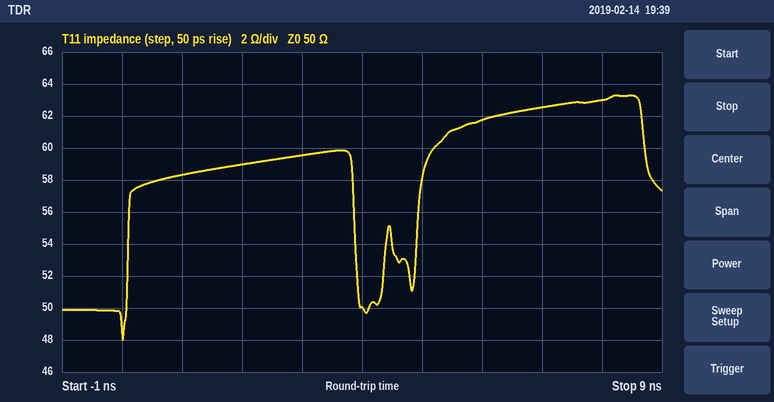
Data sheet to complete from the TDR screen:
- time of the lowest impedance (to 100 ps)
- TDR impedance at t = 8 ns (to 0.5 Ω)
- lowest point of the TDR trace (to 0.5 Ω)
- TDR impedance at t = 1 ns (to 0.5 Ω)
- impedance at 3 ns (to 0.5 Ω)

0.0 ns
63.0 Ω
48.0 Ω
58.5 Ω
59.5 Ω
